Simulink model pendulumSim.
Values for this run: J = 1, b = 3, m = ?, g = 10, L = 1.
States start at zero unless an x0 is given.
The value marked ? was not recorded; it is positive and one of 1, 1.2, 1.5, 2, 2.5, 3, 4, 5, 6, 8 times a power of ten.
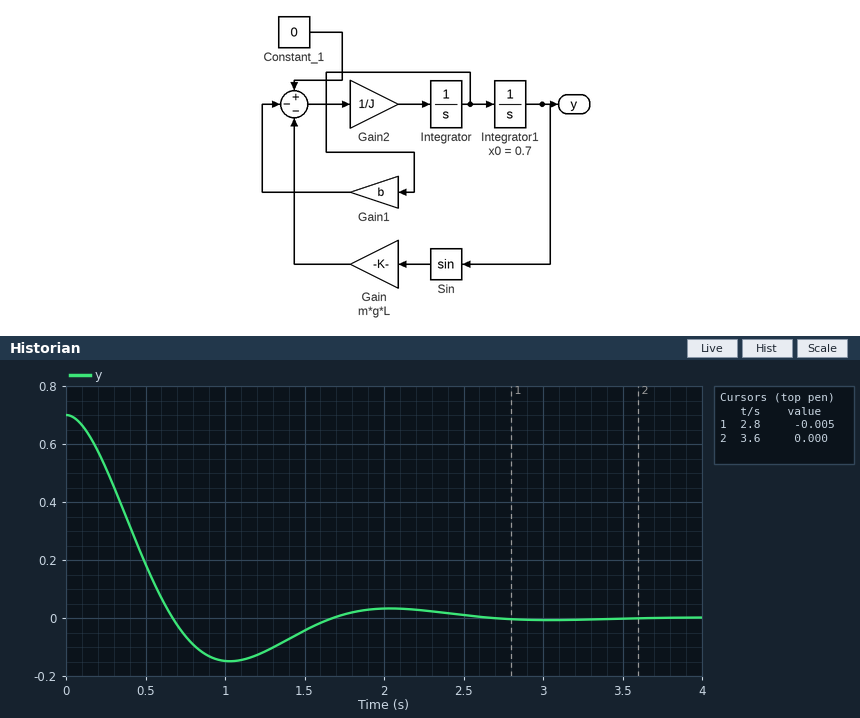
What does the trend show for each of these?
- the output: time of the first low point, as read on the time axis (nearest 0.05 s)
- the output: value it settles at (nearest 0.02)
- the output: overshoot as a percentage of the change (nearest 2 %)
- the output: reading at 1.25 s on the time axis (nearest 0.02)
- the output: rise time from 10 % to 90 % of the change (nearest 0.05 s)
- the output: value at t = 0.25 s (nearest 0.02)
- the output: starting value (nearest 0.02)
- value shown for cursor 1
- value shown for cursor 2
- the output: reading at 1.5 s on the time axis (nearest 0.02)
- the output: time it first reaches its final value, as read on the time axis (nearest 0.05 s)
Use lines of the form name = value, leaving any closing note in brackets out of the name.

the output: time of the first low point, as read on the time axis = 1.05 s
the output: value it settles at = 0.00
the output: overshoot as a percentage of the change = 22 %
the output: reading at 1.25 s on the time axis = -0.12
the output: rise time from 10 % to 90 % of the change = 0.45 s
the output: value at t = 0.25 s = 0.52
the output: starting value = 0.70
value shown for cursor 1 = -0.005
value shown for cursor 2 = 0.000
the output: reading at 1.5 s on the time axis = -0.04
the output: time it first reaches its final value, as read on the time axis = 0.65 s
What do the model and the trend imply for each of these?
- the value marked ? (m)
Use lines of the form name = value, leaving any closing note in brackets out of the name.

the value marked ? = 1.2
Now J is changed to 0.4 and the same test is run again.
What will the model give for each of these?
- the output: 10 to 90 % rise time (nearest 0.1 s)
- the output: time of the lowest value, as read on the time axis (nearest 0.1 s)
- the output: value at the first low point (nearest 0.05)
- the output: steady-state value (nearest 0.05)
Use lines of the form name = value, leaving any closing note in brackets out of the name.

the output: 10 to 90 % rise time = 0.4 s
the output: time of the lowest value, as read on the time axis = 0.8 s
the output: value at the first low point = -0.05
the output: steady-state value = 0.00
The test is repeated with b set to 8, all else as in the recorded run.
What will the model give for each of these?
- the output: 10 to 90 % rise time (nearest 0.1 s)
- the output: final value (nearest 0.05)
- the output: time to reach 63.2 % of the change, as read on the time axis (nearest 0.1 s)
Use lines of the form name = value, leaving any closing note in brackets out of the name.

the output: 10 to 90 % rise time = 1.2 s
the output: final value = 0.00
the output: time to reach 63.2 % of the change, as read on the time axis = 0.7 s
